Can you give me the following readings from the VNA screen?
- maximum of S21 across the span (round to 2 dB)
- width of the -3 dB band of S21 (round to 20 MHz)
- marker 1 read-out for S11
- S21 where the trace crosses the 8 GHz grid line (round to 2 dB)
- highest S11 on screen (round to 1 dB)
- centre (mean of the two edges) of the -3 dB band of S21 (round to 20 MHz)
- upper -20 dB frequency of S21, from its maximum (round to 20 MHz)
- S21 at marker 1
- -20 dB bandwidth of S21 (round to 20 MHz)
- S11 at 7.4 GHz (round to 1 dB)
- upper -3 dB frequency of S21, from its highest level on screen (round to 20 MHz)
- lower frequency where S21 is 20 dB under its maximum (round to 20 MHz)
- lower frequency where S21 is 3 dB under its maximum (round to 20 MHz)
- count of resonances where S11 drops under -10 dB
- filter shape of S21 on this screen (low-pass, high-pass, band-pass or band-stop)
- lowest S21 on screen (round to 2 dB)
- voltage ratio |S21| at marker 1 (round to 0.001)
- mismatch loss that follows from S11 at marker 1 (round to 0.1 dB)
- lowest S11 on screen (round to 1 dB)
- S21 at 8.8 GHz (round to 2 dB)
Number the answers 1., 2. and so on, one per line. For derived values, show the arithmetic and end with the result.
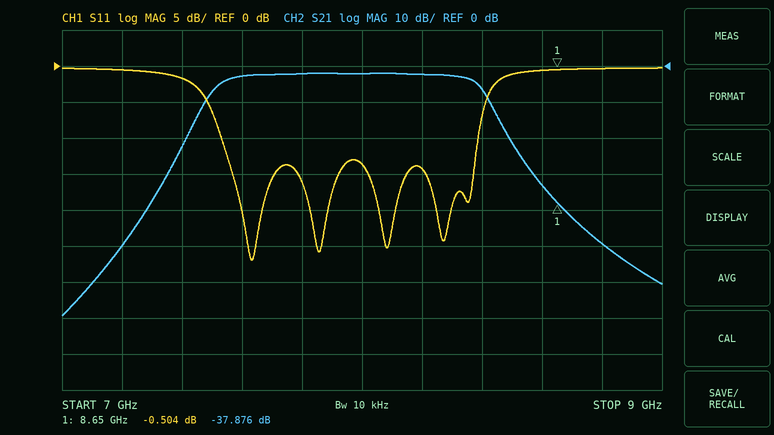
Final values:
1. -2 dB
2. 8.38 GHz − 7.52 GHz = 860 MHz
3. -0.504 dB
4. -2 dB
5. 0 dB
6. 7.96 GHz
7. 8.50 GHz
8. -37.876 dB
9. 8.50 GHz − 7.40 GHz = 1.10 GHz
10. -2 dB
11. 8.38 GHz
12. 7.40 GHz
13. 7.52 GHz
14. 4
15. band-pass
16. -70 dB
17. 10^(-37.876/20) ≈ 0.013
18. −10 log10(1 − 10^(-0.504/10)) ≈ 9.6 dB
19. -27 dB
20. -50 dB
